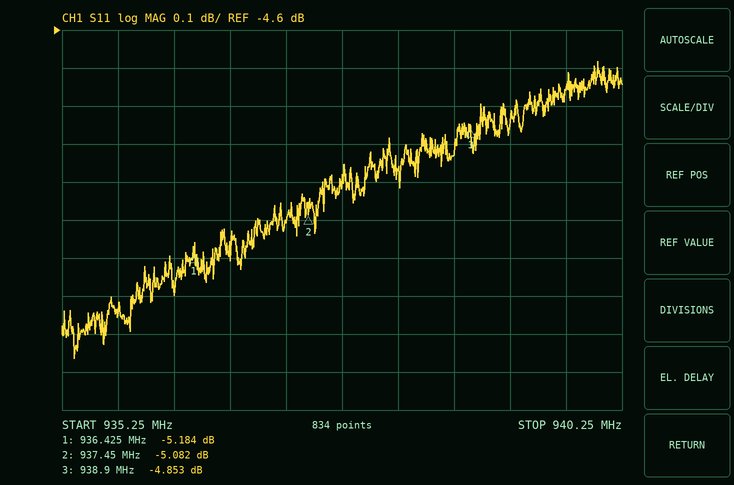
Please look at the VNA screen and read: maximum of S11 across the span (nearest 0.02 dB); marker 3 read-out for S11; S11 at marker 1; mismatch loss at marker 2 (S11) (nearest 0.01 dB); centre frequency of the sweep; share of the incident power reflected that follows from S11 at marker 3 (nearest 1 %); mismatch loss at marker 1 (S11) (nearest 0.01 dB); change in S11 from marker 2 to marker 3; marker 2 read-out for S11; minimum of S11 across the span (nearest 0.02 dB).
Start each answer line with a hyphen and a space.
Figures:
- -4.68 dB
- -4.853 dB
- -5.184 dB
- 1.61 dB
- 937.75 MHz
- 33 %
- 1.57 dB
- 0.229 dB
- -5.082 dB
- -5.46 dB
